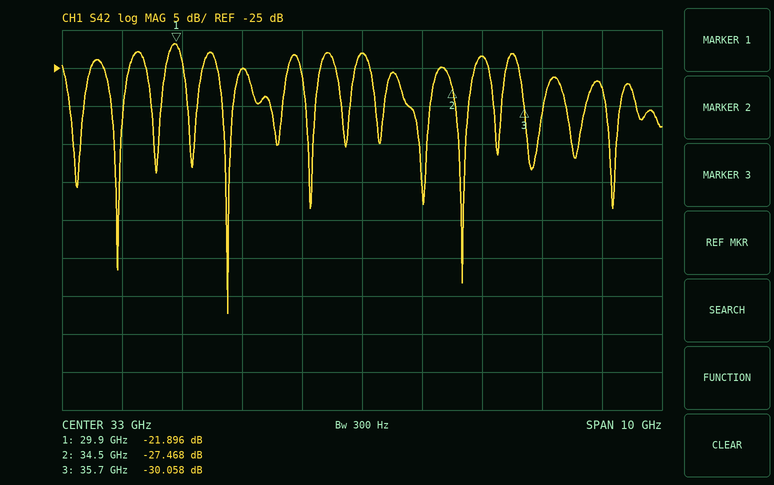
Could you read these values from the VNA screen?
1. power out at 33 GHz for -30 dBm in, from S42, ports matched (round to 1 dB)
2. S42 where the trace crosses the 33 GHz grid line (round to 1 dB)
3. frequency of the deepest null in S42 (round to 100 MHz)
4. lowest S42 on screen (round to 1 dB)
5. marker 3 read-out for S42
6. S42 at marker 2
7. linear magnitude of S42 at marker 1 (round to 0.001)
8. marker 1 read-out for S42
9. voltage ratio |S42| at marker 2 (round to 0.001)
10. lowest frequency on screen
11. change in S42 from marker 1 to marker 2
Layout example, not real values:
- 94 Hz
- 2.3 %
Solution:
- -53 dBm
- -23 dB
- 30.8 GHz
- -57 dB
- -30.058 dB
- -27.468 dB
- 0.080
- -21.896 dB
- 0.042
- 28 GHz
- -5.572 dB
